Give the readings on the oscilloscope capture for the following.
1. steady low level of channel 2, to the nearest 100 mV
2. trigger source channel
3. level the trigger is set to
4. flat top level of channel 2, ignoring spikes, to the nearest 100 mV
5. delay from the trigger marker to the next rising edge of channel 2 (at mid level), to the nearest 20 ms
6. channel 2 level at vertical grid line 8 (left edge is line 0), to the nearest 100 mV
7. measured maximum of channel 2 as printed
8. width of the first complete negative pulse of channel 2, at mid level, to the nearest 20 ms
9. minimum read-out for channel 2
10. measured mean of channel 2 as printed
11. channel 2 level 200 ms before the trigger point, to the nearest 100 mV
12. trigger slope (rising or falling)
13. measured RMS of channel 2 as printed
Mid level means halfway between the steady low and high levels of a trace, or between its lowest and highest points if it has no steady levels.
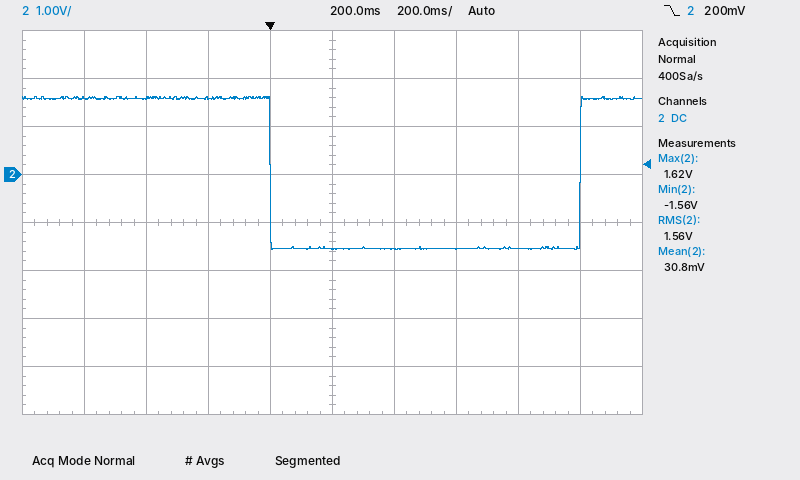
-1.5 V
channel 2
200 mV
1.6 V
1.00 s
-1.5 V
1.62 V
1.00 s
-1.56 V
30.8 mV
1.6 V
falling
1.56 V
